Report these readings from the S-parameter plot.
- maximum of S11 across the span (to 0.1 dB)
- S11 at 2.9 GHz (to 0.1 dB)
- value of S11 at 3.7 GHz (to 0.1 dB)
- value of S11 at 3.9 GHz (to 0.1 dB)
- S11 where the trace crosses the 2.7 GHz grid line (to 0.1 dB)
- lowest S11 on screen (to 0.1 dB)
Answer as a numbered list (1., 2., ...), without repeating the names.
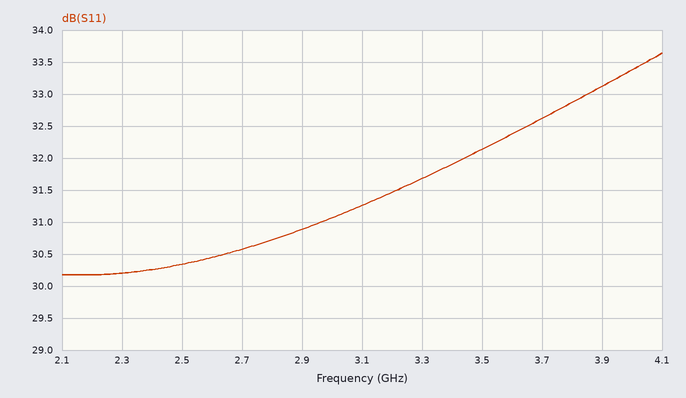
1. 33.6 dB
2. 30.9 dB
3. 32.6 dB
4. 33.1 dB
5. 30.6 dB
6. 30.2 dB
